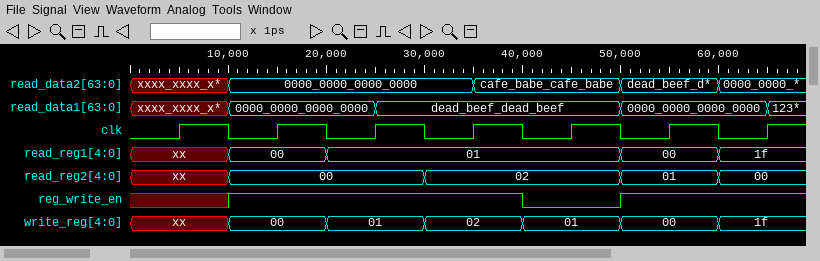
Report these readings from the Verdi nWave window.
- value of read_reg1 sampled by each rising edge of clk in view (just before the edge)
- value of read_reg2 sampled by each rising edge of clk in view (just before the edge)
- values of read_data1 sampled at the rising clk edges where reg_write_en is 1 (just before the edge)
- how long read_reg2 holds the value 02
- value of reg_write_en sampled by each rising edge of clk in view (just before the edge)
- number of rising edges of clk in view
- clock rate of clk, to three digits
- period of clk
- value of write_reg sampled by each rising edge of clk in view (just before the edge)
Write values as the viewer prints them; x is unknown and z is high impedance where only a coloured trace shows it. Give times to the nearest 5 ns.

xx, 00, 01, 01, 01, 00, 1f
xx, 00, 00, 02, 02, 01, 00
0000_0000_0000_0000, 0000_0000_0000_0000, dead_beef_dead_beef, 0000_0000_0000_0000, 0000_0000_0000_0000
20 ns
x 1 1 1 0 1 1
7
100 MHz
10 ns
xx, 00, 01, 02, 01, 00, 1f
